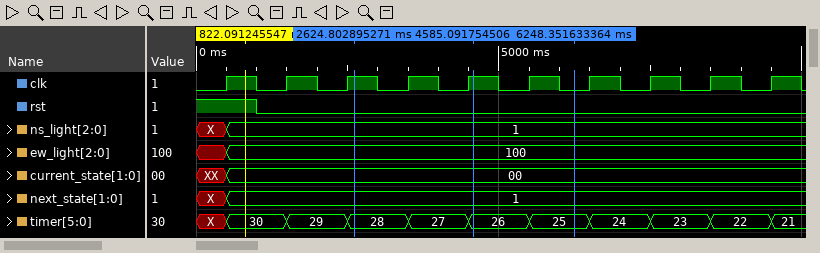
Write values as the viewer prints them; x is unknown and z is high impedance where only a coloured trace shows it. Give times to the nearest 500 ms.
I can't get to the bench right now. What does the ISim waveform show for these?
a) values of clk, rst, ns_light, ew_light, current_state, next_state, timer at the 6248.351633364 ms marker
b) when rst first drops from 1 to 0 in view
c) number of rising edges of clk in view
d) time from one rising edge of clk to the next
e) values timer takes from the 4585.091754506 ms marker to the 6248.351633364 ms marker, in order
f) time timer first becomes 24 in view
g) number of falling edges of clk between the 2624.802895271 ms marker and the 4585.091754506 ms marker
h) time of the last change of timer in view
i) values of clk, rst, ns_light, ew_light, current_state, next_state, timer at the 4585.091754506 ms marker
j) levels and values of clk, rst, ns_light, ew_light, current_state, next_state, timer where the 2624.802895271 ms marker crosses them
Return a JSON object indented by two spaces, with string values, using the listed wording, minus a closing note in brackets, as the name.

{
  "values of clk, rst, ns_light, ew_light, current_state, next_state, timer at the 6248.351633364 ms marker": "clk=0, rst=0, ns_light=1, ew_light=100, current_state=00, next_state=1, timer=25",
  "when rst first drops from 1 to 0 in view": "1000 ms",
  "number of rising edges of clk in view": "10",
  "time from one rising edge of clk to the next": "1000 ms",
  "values timer takes from the 4585.091754506 ms marker to the 6248.351633364 ms marker, in order": "26, 25",
  "time timer first becomes 24 in view": "6500 ms",
  "number of falling edges of clk between the 2624.802895271 ms marker and the 4585.091754506 ms marker": "2",
  "time of the last change of timer in view": "9500 ms",
  "values of clk, rst, ns_light, ew_light, current_state, next_state, timer at the 4585.091754506 ms marker": "clk=1, rst=0, ns_light=1, ew_light=100, current_state=00, next_state=1, timer=26",
  "levels and values of clk, rst, ns_light, ew_light, current_state, next_state, timer where the 2624.802895271 ms marker crosses them": "clk=1, rst=0, ns_light=1, ew_light=100, current_state=00, next_state=1, timer=28"
}
